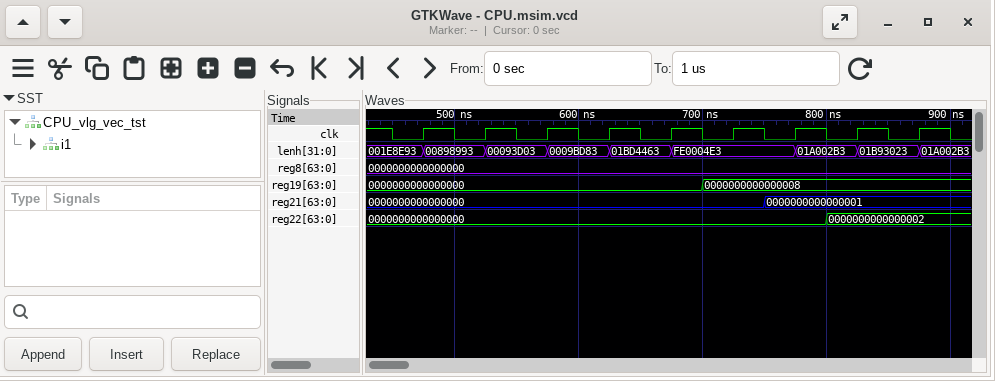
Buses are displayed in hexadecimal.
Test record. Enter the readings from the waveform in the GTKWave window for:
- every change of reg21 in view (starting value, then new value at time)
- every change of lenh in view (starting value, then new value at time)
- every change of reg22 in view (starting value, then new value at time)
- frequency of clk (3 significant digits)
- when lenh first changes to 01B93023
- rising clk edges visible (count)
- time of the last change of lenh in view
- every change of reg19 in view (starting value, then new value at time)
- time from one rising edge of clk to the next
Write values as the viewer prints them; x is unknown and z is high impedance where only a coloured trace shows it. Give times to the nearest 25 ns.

0000000000000000, 0000000000000001 at 750 ns
001E8E93, 00898993 at 475 ns, 00093D03 at 525 ns, 0009BD83 at 575 ns, 01BD4463 at 625 ns, FE0004E3 at 675 ns, 01A002B3 at 775 ns, 01B93023 at 825 ns, 01A002B3 at 875 ns
0000000000000000, 0000000000000002 at 800 ns
20.0 MHz
825 ns
9
875 ns
0000000000000000, 0000000000000008 at 700 ns
50 ns
